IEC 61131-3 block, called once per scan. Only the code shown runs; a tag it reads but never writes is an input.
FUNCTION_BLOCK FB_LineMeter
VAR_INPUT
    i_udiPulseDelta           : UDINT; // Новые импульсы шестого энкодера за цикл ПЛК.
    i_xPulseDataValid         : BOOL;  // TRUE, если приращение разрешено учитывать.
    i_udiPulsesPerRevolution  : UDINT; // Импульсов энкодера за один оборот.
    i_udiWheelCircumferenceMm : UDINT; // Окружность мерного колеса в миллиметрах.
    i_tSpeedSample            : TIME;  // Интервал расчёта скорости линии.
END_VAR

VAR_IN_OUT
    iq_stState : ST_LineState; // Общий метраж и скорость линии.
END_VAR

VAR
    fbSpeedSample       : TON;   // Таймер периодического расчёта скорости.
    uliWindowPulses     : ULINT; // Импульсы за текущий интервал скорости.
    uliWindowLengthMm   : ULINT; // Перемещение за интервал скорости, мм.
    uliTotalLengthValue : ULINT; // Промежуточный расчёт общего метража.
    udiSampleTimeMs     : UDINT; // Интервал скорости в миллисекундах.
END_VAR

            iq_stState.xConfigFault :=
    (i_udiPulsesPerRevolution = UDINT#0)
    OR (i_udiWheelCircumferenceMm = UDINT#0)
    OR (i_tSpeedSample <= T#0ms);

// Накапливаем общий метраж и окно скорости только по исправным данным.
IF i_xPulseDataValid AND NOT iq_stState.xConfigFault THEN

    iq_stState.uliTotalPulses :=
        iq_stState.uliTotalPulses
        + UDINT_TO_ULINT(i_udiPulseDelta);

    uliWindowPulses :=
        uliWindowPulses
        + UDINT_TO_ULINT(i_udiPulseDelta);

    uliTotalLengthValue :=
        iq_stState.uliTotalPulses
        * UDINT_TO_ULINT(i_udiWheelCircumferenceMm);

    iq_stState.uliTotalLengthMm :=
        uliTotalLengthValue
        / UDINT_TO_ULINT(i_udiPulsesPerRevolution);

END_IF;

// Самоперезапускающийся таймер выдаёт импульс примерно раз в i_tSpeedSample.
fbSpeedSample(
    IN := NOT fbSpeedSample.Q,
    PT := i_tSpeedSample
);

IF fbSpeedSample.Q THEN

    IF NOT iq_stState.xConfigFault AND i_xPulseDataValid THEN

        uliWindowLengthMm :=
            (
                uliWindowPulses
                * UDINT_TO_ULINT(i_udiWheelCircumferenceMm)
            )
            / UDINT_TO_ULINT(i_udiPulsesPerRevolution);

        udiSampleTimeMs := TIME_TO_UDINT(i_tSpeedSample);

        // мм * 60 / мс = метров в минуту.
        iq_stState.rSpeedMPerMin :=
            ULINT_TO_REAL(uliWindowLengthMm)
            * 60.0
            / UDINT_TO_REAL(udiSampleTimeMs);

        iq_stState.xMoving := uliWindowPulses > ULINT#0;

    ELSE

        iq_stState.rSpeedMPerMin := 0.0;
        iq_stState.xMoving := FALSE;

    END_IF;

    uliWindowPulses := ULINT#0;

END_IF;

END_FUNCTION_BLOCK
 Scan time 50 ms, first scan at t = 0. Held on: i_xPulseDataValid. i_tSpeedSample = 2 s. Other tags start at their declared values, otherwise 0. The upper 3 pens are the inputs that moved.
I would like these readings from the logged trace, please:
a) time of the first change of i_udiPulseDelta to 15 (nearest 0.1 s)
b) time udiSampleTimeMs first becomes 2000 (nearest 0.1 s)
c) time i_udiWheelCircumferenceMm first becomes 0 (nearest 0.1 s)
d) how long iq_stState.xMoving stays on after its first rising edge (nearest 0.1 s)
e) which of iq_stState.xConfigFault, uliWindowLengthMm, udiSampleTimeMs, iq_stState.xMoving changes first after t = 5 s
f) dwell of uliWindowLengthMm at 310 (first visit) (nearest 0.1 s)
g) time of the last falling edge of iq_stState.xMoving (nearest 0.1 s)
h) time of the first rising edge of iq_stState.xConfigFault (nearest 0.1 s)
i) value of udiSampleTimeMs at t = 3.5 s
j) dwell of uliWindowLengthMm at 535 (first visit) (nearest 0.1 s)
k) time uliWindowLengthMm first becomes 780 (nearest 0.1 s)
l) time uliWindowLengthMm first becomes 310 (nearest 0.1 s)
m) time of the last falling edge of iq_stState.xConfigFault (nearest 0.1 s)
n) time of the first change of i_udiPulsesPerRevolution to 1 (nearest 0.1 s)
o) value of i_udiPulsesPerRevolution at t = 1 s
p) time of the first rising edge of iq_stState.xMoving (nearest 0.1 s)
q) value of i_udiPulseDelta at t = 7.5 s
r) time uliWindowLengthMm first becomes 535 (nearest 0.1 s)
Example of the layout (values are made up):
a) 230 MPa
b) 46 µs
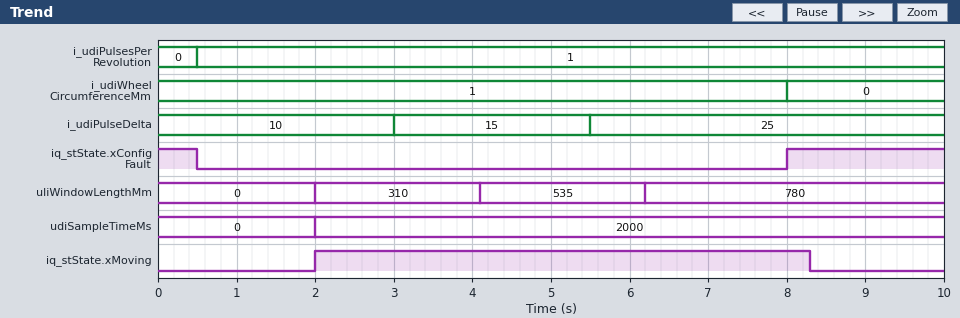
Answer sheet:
a) 3.0 s
b) 2.0 s
c) 8.0 s
d) 6.3 s
e) uliWindowLengthMm
f) 2.1 s
g) 8.3 s
h) 8.0 s
i) 2000
j) 2.1 s
k) 6.2 s
l) 2.0 s
m) 0.5 s
n) 0.5 s
o) 1
p) 2.0 s
q) 25
r) 4.1 s
